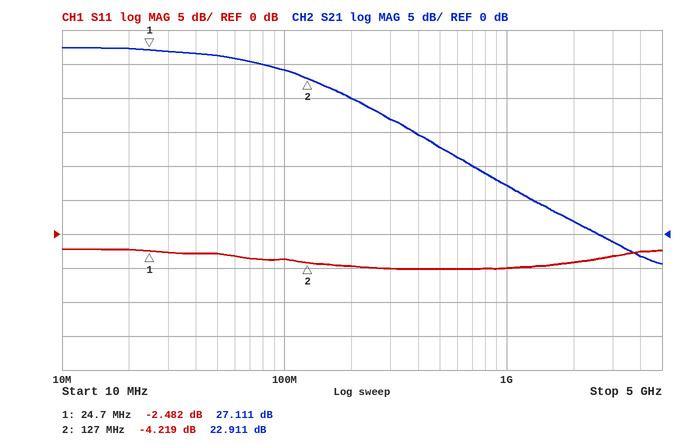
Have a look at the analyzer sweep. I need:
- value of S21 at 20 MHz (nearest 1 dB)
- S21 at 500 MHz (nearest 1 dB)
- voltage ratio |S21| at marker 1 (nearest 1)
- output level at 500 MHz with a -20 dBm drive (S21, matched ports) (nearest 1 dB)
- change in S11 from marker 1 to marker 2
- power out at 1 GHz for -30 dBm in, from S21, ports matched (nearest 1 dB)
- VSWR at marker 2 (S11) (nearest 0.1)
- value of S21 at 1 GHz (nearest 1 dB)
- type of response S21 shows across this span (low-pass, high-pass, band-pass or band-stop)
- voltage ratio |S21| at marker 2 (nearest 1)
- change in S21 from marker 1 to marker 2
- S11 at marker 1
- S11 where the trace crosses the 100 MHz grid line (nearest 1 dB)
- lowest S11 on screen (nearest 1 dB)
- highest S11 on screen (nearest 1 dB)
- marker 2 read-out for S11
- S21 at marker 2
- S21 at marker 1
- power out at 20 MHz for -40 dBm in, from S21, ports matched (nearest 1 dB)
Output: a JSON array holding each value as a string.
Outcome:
["27 dB", "13 dB", "23", "-7 dBm", "-1.737 dB", "-23 dBm", "4.2", "7 dB", "low-pass", "14", "-4.200 dB", "-2.482 dB", "-4 dB", "-5 dB", "-2 dB", "-4.219 dB", "22.911 dB", "27.111 dB", "-13 dBm"]
